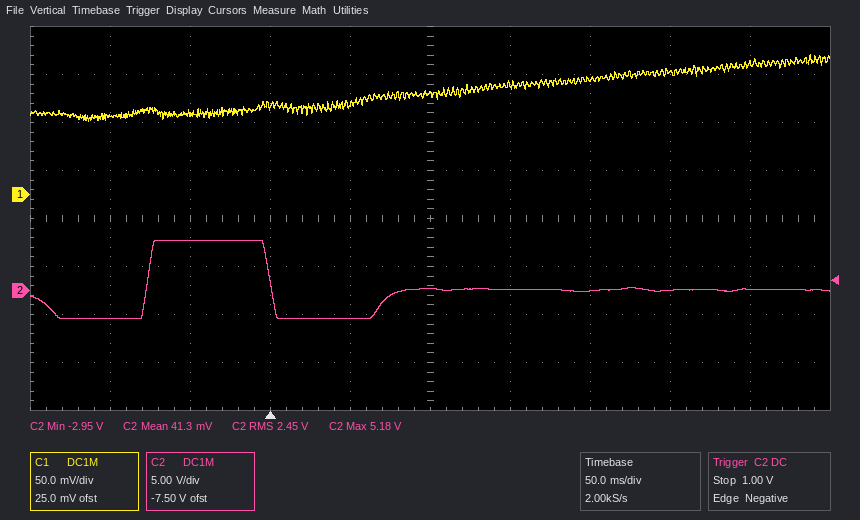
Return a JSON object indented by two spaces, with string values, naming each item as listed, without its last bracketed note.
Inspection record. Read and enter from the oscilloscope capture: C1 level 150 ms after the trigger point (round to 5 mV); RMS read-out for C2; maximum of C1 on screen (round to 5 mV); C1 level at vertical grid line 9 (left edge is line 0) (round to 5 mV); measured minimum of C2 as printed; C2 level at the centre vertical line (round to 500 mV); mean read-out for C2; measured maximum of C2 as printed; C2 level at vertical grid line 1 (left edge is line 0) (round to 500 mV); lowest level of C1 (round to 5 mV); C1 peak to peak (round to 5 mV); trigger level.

{
  "C1 level 150 ms after the trigger point": "115 mV",
  "RMS read-out for C2": "2.45 V",
  "maximum of C1 on screen": "145 mV",
  "C1 level at vertical grid line 9 (left edge is line 0)": "135 mV",
  "measured minimum of C2 as printed": "-2.95 V",
  "C2 level at the centre vertical line": "0.0 V",
  "mean read-out for C2": "41.3 mV",
  "measured maximum of C2 as printed": "5.18 V",
  "C2 level at vertical grid line 1 (left edge is line 0)": "-3.0 V",
  "lowest level of C1": "75 mV",
  "C1 peak to peak": "70 mV",
  "trigger level": "1.00 V"
}
